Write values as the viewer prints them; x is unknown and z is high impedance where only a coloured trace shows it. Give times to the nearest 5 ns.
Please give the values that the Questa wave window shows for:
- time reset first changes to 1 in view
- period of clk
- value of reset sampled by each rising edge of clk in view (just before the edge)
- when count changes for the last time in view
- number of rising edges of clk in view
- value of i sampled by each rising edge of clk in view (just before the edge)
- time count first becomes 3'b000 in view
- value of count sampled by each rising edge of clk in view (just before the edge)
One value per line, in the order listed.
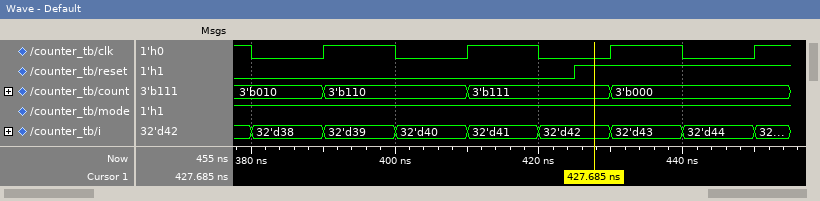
425 ns
20 ns
0 0 1 1
430 ns
4
32'd38, 32'd40, 32'd42, 32'd44
430 ns
3'b010, 3'b110, 3'b111, 3'b000
